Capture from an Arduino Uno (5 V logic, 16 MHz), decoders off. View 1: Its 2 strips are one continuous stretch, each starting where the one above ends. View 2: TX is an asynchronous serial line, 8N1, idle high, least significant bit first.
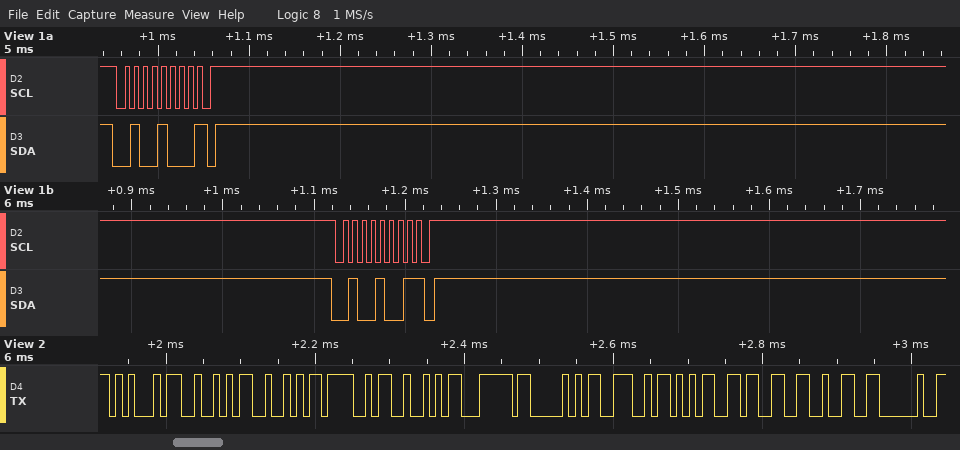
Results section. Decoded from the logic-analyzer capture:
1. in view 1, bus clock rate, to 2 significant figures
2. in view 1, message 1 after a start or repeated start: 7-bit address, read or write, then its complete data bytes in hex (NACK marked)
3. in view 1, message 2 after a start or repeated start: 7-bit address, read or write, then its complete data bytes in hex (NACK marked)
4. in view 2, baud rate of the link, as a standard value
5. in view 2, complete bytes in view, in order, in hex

100 kHz
0x24 write NACK
0x24 read NACK
115200 baud
0x45 0x52 0x52 0x4F 0x52 0x7C 0x50 0x4E 0x35 0x33 0x32 0x20
